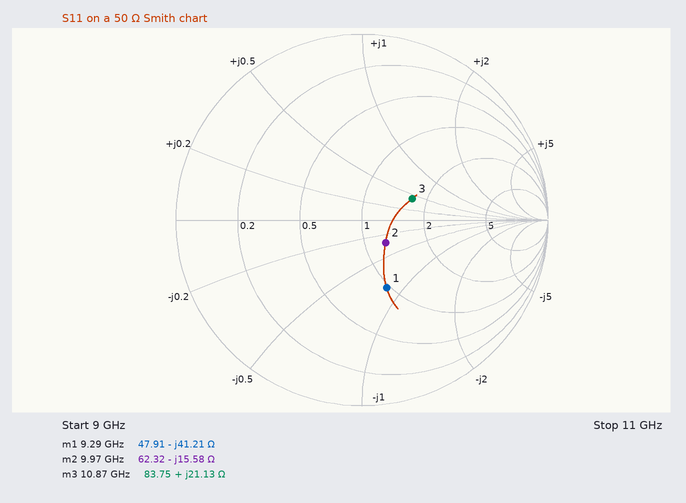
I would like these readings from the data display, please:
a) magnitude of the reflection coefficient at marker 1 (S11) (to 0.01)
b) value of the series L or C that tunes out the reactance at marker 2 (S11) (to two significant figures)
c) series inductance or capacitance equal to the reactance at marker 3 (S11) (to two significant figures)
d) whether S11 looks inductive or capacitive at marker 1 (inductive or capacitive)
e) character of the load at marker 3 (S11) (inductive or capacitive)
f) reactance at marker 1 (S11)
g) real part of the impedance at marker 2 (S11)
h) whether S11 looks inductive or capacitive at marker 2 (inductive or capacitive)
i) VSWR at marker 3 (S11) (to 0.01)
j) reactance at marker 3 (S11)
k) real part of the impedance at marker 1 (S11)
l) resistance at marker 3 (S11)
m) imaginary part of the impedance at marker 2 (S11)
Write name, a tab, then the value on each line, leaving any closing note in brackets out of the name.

magnitude of the reflection coefficient at marker 1 (S11)	0.39
value of the series L or C that tunes out the reactance at marker 2 (S11)	250 pH
series inductance or capacitance equal to the reactance at marker 3 (S11)	310 pH
whether S11 looks inductive or capacitive at marker 1	capacitive
character of the load at marker 3 (S11)	inductive
reactance at marker 1	-41.21 Ω
real part of the impedance at marker 2	62.32 Ω
whether S11 looks inductive or capacitive at marker 2	capacitive
VSWR at marker 3 (S11)	1.83
reactance at marker 3	+21.13 Ω
real part of the impedance at marker 1	47.91 Ω
resistance at marker 3	83.75 Ω
imaginary part of the impedance at marker 2	-15.58 Ω
